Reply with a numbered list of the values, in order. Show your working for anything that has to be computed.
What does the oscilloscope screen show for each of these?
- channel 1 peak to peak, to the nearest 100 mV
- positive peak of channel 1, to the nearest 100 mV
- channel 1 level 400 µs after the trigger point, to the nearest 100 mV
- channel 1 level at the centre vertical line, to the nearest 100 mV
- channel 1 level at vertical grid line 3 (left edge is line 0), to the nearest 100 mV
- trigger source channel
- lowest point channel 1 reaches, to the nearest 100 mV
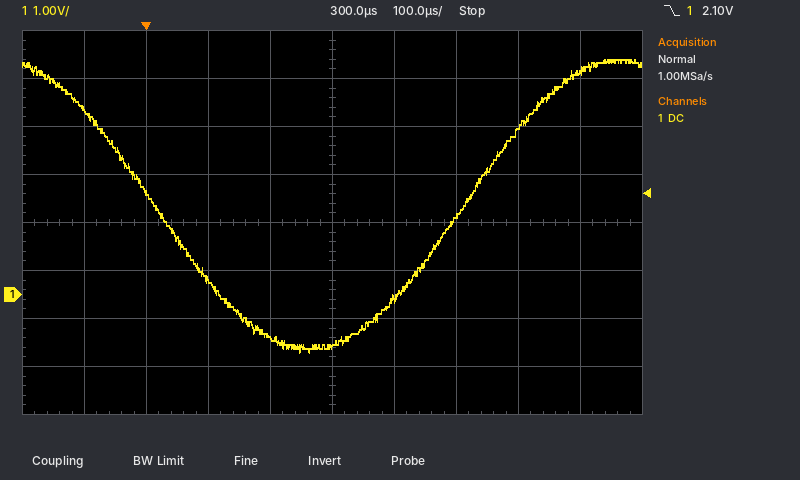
1. 4.9 V − (-1.2 V) = 6.1 V
2. 4.9 V
3. -100 mV
4. -1.1 V
5. 300 mV
6. channel 1
7. -1.2 V
